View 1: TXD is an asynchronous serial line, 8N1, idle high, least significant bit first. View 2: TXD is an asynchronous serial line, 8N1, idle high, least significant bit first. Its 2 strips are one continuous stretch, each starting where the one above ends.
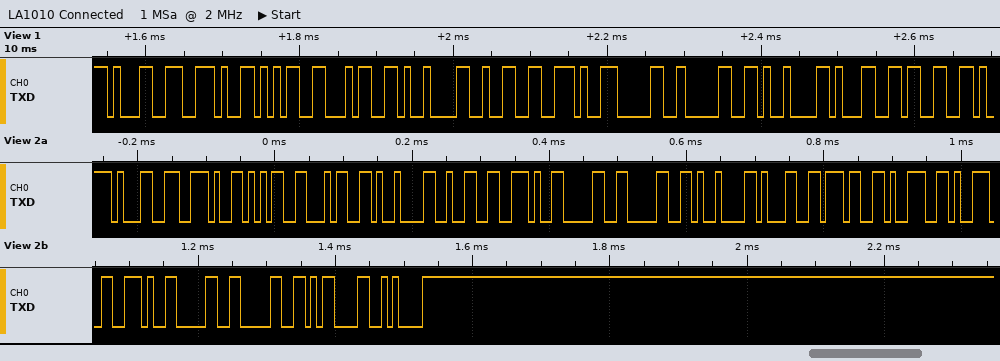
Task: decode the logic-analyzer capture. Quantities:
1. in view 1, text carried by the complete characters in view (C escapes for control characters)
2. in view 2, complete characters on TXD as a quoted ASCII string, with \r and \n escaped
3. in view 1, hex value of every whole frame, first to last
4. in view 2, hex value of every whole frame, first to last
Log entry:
"1.54\t2.00\t13"
"1.54\t2.00\t1799.00\r\n"
31 2E 35 34 09 32 2E 30 30 09 31 33
31 2E 35 34 09 32 2E 30 30 09 31 37 39 39 2E 30 30 0D 0A
